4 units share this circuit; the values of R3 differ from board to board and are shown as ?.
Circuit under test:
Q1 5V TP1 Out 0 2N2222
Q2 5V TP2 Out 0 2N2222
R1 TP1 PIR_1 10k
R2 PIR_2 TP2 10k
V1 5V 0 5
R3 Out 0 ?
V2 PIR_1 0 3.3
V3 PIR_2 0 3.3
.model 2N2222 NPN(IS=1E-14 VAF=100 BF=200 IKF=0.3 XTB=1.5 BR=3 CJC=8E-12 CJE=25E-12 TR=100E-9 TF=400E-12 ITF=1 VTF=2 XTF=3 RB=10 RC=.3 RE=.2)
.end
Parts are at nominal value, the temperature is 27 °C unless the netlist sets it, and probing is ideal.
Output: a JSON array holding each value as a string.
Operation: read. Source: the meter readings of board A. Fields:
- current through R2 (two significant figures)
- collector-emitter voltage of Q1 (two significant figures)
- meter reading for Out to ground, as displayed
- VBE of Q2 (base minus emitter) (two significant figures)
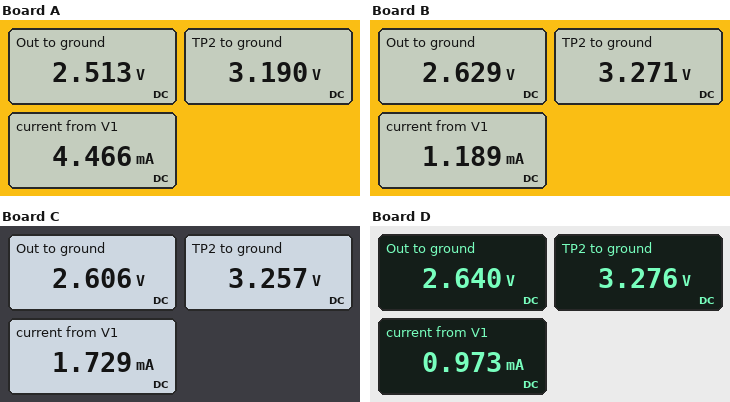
["11 µA", "2.5 V", "2.513 V", "680 mV"]
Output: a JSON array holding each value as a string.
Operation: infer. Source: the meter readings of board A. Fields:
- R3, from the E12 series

["560 Ω"]
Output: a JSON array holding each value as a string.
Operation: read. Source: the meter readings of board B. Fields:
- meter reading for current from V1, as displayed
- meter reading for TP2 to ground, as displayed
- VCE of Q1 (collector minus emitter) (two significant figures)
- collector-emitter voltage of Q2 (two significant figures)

["1.189 mA", "3.271 V", "2.4 V", "2.4 V"]
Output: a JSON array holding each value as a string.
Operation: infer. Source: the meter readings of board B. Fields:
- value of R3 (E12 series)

["2.2 kΩ"]
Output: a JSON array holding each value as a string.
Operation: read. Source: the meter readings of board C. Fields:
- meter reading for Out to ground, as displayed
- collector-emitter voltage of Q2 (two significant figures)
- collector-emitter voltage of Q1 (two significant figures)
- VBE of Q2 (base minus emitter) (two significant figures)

["2.606 V", "2.4 V", "2.4 V", "650 mV"]
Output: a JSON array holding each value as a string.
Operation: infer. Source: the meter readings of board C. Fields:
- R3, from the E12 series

["1.5 kΩ"]
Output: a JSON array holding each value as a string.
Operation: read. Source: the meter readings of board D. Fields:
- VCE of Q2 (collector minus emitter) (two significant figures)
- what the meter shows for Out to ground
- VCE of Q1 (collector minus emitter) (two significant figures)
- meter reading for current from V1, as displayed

["2.4 V", "2.640 V", "2.4 V", "0.973 mA"]
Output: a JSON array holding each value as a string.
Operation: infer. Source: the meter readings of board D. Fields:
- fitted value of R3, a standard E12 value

["2.7 kΩ"]
